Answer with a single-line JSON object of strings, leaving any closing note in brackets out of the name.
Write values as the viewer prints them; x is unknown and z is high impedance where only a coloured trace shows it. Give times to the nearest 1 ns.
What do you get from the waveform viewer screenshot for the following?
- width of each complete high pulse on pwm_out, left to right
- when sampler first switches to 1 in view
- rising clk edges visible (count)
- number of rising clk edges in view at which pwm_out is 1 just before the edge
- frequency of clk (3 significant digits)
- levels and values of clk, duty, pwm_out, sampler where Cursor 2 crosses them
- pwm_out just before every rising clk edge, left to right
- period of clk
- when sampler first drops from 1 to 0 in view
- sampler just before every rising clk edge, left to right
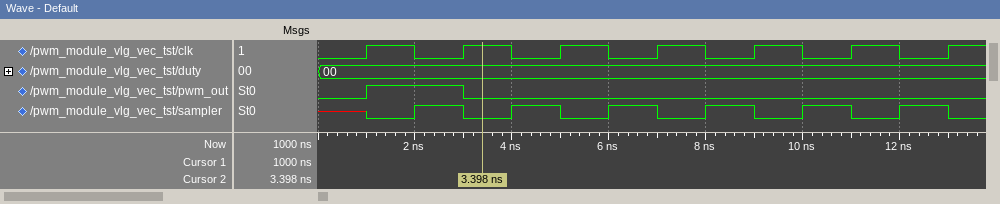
{"width of each complete high pulse on pwm_out, left to right": "2 ns", "when sampler first switches to 1 in view": "2 ns", "rising clk edges visible": "7", "number of rising clk edges in view at which pwm_out is 1 just before the edge": "1", "frequency of clk": "500 MHz", "levels and values of clk, duty, pwm_out, sampler where Cursor 2 crosses them": "clk=1, duty=00, pwm_out=0, sampler=0", "pwm_out just before every rising clk edge, left to right": "0 1 0 0 0 0 0", "period of clk": "2 ns", "when sampler first drops from 1 to 0 in view": "3 ns", "sampler just before every rising clk edge, left to right": "x 1 1 1 1 1 1"}
